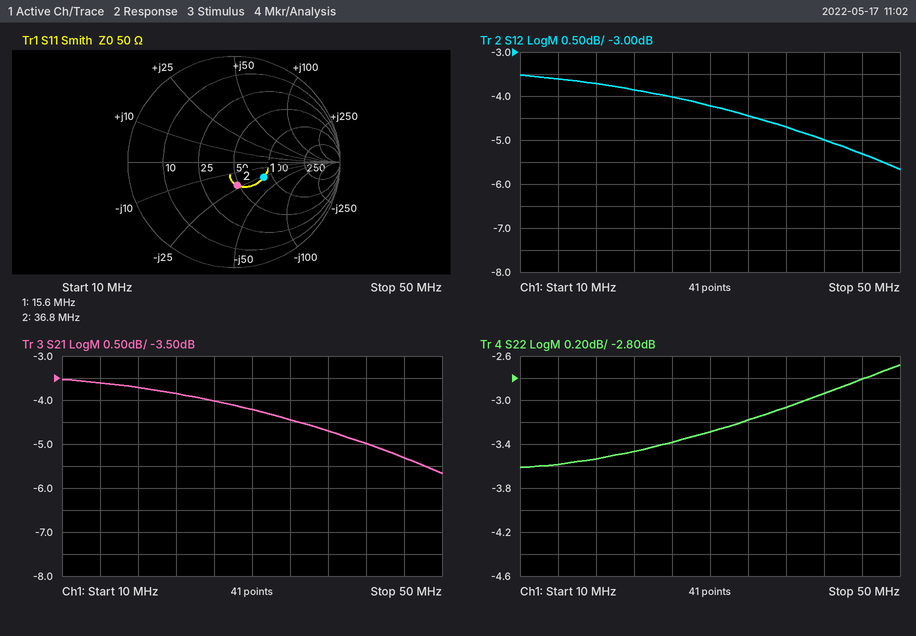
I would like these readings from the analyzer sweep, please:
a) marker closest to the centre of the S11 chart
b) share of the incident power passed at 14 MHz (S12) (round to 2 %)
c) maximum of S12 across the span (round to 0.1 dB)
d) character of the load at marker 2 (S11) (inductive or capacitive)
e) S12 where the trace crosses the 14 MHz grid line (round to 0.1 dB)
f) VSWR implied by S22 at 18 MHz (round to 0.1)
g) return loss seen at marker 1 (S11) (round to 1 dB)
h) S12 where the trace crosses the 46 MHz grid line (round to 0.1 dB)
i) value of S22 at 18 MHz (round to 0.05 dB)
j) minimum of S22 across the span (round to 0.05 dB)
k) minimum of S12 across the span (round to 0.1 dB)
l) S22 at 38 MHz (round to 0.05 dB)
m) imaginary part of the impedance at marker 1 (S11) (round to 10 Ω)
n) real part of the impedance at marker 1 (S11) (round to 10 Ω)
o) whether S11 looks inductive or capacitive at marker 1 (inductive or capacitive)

marker 2
44 %
-3.5 dB
capacitive
-3.6 dB
5.0
10 dB
-5.3 dB
-3.55 dB
-3.60 dB
-5.7 dB
-3.05 dB
-30 Ω
80 Ω
capacitive
